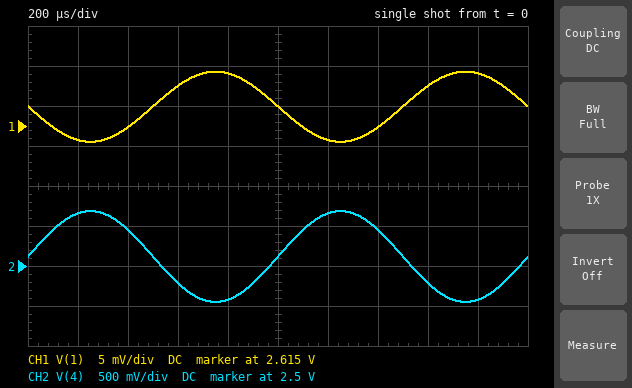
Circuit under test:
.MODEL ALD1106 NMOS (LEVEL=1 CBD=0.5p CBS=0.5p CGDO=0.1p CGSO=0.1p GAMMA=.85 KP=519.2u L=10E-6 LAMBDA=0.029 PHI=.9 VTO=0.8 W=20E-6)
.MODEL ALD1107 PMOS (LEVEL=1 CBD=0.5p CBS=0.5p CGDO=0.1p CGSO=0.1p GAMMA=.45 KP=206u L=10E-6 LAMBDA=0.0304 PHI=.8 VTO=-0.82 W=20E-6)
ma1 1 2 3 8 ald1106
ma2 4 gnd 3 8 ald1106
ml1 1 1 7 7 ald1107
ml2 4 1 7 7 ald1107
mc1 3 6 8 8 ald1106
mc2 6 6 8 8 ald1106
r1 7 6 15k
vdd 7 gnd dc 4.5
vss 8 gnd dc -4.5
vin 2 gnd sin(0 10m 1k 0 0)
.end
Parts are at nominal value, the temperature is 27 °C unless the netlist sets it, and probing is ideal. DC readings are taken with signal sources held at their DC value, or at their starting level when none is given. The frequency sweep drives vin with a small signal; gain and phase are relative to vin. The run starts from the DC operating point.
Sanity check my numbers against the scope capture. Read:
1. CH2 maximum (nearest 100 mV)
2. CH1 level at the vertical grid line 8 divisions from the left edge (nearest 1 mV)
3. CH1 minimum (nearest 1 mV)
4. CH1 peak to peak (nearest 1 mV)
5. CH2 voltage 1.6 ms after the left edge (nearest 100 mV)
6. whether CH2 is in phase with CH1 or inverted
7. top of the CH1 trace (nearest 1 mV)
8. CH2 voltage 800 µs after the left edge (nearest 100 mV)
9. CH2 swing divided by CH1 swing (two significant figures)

3.2 V
2.620 V
2.613 V
9 mV
2.3 V
inverted
2.622 V
2.1 V
130
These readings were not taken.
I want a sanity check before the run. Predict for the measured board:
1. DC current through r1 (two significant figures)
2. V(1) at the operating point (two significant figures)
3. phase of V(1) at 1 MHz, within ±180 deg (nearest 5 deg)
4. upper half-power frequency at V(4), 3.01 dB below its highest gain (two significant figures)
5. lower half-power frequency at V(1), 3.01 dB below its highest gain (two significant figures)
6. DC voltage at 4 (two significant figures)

480 µA
2.6 V
-170 deg
4.9 MHz
3.1 MHz
2.6 V
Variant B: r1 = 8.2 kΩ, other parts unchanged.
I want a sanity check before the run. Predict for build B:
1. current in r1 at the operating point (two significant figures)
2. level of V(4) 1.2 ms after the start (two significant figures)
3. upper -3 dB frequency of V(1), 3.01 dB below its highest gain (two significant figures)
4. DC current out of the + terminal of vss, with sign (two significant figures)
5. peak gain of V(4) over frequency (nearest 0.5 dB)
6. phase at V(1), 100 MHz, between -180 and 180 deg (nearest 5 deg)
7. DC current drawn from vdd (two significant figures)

850 µA
2.7 V
440 MHz
-1.7 mA
32.5 dB
170 deg
1.7 mA
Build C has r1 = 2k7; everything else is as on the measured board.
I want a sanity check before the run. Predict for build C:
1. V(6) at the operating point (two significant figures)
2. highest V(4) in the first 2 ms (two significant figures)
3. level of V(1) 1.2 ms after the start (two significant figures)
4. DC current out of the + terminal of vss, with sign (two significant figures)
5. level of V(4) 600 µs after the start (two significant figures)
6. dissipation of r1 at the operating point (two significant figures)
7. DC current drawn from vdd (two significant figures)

-1.7 V
1.7 V
1.5 V
-4.5 mA
1.3 V
14 mW
4.5 mA
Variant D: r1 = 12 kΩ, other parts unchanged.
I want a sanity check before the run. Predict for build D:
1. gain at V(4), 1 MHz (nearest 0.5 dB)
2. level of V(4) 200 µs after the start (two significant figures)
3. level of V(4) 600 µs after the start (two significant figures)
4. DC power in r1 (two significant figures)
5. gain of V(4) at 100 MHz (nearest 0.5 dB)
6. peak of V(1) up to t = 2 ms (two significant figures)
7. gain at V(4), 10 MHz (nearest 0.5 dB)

34.0 dB
3.0 V
2.2 V
4.3 mW
9.5 dB
2.5 V
28.5 dB
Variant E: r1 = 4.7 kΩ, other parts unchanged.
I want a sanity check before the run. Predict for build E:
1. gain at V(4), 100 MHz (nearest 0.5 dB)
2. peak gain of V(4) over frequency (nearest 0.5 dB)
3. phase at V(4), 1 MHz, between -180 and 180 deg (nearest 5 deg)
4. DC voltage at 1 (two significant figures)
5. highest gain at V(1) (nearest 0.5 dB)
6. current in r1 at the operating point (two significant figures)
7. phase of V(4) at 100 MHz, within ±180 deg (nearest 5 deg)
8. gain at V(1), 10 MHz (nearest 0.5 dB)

13.5 dB
30.5 dB
-5 deg
1.9 V
-2.0 dB
1.4 mA
-90 deg
-4.5 dB
